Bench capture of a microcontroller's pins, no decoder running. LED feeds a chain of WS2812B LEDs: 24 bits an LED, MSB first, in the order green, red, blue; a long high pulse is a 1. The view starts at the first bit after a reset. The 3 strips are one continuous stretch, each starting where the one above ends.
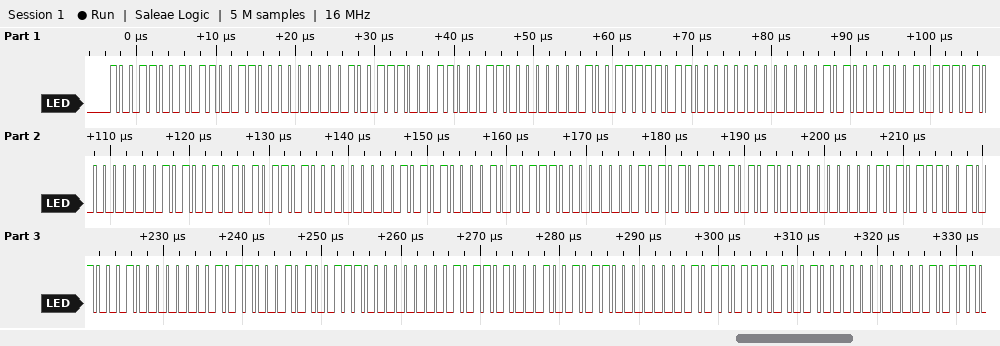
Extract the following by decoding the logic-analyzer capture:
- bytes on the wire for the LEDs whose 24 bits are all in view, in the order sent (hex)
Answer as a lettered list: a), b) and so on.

a) 99 66 00 9C 63 00 9F 60 00 A2 5D 00 A5 5A 00 A8 57 00 AB 54 00 AE 51 00 B1 4E 00 B4 4B 00 B7 48 00
